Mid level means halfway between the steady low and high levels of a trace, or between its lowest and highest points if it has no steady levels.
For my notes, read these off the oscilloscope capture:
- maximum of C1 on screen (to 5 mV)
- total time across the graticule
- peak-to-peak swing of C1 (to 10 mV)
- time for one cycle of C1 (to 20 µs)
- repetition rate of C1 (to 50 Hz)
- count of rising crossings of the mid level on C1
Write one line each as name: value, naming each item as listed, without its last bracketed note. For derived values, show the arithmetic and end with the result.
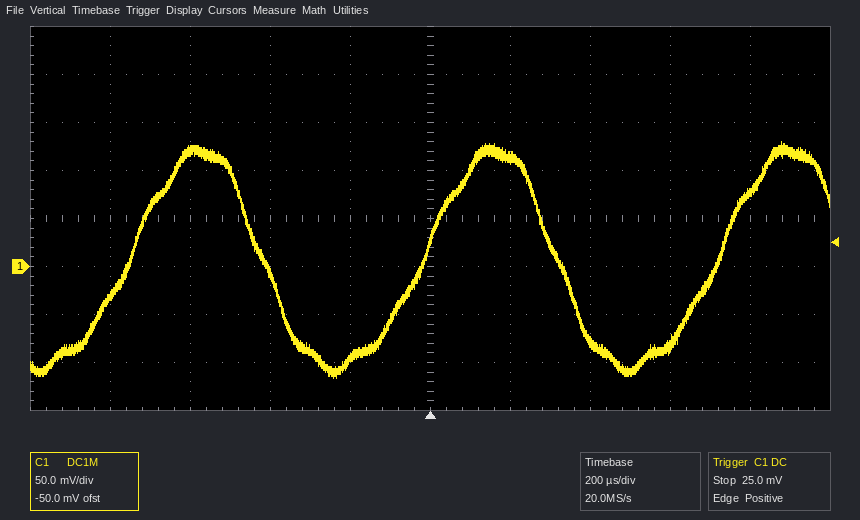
maximum of C1 on screen: 130 mV
total time across the graticule: 2 ms
peak-to-peak swing of C1: 250 mV
time for one cycle of C1: 740 µs
repetition rate of C1: 1 / 740 µs ≈ 1.35 kHz
count of rising crossings of the mid level on C1: 3
